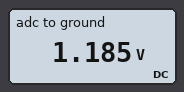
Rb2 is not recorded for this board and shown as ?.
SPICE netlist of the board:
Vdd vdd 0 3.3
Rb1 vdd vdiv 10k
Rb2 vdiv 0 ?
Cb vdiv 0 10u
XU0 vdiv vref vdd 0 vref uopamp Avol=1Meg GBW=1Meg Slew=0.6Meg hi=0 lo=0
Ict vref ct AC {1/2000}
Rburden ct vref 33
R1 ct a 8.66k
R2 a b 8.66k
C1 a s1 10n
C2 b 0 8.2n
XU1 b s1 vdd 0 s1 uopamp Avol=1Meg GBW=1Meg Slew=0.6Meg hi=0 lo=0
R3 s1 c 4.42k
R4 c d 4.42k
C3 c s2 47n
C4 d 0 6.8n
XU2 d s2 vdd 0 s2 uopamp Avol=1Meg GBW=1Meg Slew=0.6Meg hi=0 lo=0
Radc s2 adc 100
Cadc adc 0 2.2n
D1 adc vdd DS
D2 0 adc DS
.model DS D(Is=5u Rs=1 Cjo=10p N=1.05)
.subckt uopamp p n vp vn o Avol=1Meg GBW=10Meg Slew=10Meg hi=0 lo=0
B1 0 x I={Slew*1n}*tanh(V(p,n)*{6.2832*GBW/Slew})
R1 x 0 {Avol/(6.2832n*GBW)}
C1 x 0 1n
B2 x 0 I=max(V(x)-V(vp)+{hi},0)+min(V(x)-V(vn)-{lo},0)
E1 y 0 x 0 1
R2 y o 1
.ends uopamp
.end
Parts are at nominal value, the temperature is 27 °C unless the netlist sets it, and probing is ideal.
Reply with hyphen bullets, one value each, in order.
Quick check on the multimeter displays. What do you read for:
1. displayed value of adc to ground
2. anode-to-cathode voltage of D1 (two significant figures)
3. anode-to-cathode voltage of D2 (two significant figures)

- 1.185 V
- -2.1 V
- -1.2 V
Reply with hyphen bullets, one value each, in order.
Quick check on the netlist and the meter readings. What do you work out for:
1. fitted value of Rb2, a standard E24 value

- 5.6 kΩ
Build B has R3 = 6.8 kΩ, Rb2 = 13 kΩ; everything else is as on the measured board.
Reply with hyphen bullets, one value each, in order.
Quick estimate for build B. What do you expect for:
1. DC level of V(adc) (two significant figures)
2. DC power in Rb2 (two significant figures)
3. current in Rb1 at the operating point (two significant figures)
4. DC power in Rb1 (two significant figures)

- 1.9 V
- 270 µW
- 140 µA
- 210 µW
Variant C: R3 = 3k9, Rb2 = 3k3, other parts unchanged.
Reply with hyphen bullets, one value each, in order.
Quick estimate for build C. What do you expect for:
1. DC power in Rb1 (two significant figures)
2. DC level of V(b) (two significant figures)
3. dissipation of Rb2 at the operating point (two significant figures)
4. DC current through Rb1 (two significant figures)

- 620 µW
- 820 mV
- 200 µW
- 250 µA
